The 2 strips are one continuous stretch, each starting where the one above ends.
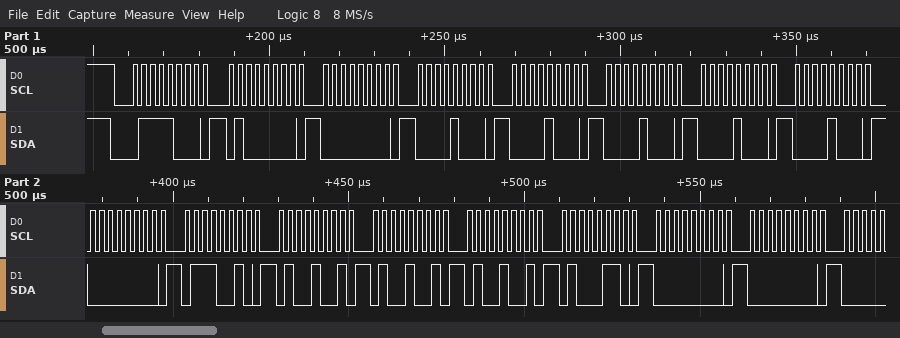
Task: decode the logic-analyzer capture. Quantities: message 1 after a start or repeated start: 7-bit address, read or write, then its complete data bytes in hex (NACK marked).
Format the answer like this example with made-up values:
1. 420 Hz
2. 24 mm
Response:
1. 0x3C write: 40 00 08 08 08 08 08 00 72 49 49 49 46 00 00
